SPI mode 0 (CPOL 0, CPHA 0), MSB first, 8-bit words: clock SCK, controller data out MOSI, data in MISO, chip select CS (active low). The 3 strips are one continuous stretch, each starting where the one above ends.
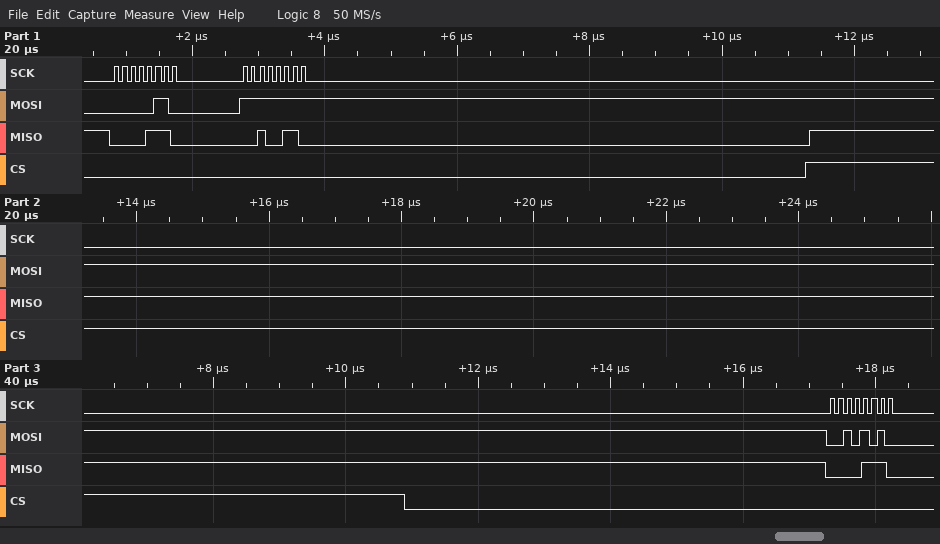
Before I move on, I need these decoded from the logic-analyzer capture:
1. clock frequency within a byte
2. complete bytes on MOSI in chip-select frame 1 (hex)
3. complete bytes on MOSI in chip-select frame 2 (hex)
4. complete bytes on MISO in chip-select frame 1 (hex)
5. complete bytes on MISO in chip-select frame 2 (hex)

8 MHz
06 FF
2A
0E 26
0E
